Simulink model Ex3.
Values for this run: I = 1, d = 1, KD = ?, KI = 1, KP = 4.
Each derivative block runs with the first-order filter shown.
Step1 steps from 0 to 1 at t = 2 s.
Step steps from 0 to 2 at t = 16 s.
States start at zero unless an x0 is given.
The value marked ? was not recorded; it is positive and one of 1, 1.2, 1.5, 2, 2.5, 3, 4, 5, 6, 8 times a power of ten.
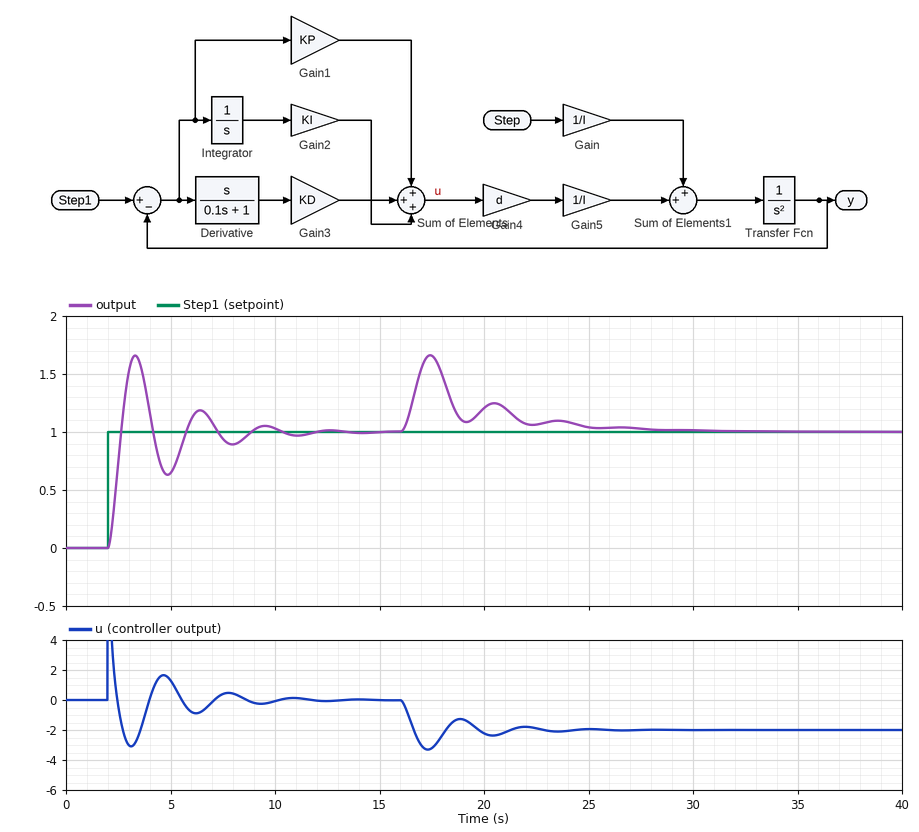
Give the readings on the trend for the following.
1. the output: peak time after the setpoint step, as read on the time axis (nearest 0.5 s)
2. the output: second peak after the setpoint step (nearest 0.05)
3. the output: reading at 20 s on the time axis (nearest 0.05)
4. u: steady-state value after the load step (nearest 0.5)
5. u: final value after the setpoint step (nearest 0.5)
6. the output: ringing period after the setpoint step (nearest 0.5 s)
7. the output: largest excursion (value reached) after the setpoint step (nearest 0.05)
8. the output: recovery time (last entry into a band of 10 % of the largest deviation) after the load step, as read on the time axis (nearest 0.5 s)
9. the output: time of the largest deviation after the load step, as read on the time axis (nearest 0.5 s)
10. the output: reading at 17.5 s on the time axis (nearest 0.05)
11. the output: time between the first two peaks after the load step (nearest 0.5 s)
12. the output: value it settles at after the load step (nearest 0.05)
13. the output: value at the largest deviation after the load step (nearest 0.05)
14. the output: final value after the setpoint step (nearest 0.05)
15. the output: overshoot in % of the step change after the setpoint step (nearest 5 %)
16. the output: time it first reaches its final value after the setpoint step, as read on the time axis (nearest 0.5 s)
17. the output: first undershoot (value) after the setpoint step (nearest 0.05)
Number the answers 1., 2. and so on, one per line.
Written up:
1. 3.5 s
2. 1.20
3. 1.20
4. -2.0
5. 0.0
6. 3.0 s
7. 1.65
8. 24.5 s
9. 17.5 s
10. 1.65
11. 3.0 s
12. 1.00
13. 1.65
14. 1.00
15. 65 %
16. 2.5 s
17. 0.65
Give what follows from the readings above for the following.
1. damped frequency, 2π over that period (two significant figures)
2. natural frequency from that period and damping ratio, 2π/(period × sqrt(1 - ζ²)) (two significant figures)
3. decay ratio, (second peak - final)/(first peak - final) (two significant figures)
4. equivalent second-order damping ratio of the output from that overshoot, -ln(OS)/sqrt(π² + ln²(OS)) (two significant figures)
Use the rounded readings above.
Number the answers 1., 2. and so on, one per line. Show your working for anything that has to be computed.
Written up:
1. 2π / 3 = 2.1 rad/s
2. 2π / (3 × sqrt(1 - 0.14²)) = 2.1 rad/s
3. (1.2 - 1) / (1.65 - 1) = 0.31
4. ln(0.65) = -0.431; 0.431 / sqrt(9.870 + 0.186) = 0.14
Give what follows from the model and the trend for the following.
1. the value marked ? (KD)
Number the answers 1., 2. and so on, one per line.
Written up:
1. 1
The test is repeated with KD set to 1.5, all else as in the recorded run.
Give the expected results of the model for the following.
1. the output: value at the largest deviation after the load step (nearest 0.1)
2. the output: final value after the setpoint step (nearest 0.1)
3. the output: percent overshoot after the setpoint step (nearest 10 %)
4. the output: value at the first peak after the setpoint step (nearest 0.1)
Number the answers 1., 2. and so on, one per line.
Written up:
1. 1.6
2. 1.0
3. 50 %
4. 1.5
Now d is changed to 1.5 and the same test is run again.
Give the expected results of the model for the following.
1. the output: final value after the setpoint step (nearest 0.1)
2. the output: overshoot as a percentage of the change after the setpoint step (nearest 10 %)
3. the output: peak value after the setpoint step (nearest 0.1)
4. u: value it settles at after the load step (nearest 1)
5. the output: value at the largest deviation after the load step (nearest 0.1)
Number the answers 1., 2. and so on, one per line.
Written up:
1. 1.0
2. 60 %
3. 1.6
4. -1
5. 1.4
